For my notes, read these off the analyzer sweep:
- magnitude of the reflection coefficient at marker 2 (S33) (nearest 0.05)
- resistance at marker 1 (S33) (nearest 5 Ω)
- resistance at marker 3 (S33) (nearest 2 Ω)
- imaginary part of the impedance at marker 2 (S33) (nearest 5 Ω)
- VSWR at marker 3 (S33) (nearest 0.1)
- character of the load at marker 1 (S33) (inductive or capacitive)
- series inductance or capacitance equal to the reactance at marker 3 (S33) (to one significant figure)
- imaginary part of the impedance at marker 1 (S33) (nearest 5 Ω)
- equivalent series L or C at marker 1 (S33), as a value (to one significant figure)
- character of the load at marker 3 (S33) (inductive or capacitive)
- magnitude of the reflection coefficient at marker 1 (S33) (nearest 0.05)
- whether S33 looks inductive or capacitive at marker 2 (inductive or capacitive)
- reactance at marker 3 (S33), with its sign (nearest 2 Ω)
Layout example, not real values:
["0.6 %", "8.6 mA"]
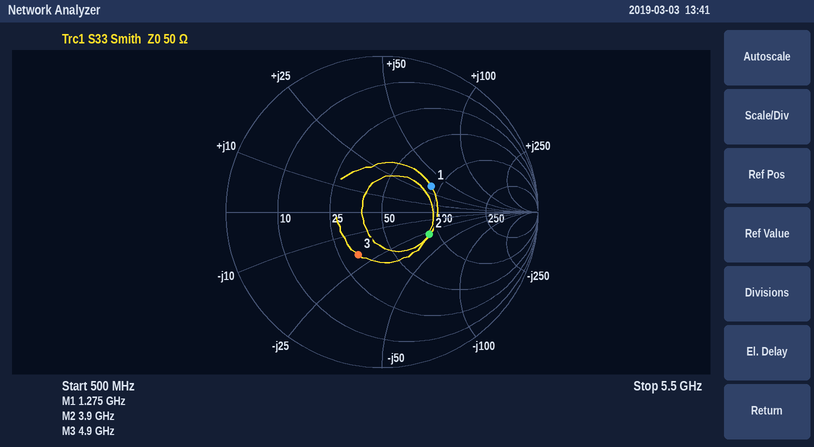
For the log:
["0.35", "90 Ω", "32 Ω", "-30 Ω", "1.9", "inductive", "2 pF", "+35 Ω", "4 nH", "capacitive", "0.35", "capacitive", "-20 Ω"]
